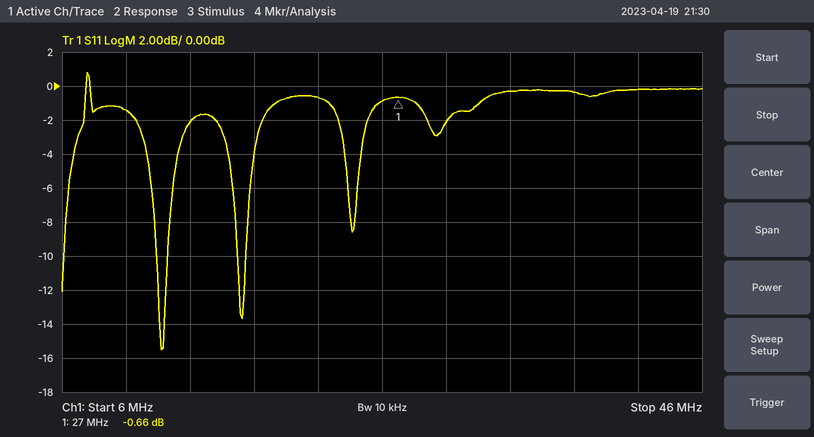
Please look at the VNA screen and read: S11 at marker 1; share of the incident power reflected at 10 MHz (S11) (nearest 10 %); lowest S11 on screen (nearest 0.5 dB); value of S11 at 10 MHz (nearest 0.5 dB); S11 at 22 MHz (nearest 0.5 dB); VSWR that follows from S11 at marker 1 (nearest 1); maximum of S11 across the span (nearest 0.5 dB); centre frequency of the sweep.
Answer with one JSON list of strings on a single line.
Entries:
["-0.66 dB", "70 %", "-15.5 dB", "-1.5 dB", "-0.5 dB", "26", "1.0 dB", "26 MHz"]
